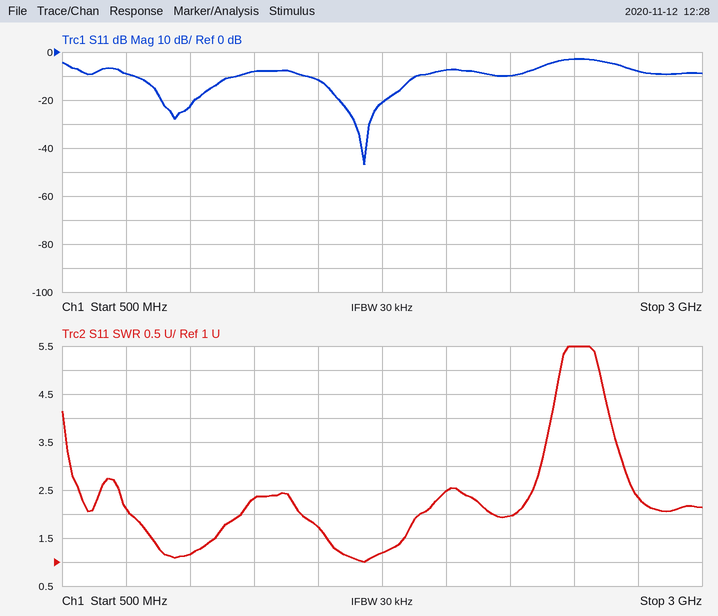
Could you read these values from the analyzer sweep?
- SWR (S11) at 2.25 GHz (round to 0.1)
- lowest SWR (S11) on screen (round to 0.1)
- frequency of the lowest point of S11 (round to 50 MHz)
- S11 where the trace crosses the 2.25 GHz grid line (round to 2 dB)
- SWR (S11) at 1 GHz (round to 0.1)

2.0
1.0
1.70 GHz
-10 dB
1.2
